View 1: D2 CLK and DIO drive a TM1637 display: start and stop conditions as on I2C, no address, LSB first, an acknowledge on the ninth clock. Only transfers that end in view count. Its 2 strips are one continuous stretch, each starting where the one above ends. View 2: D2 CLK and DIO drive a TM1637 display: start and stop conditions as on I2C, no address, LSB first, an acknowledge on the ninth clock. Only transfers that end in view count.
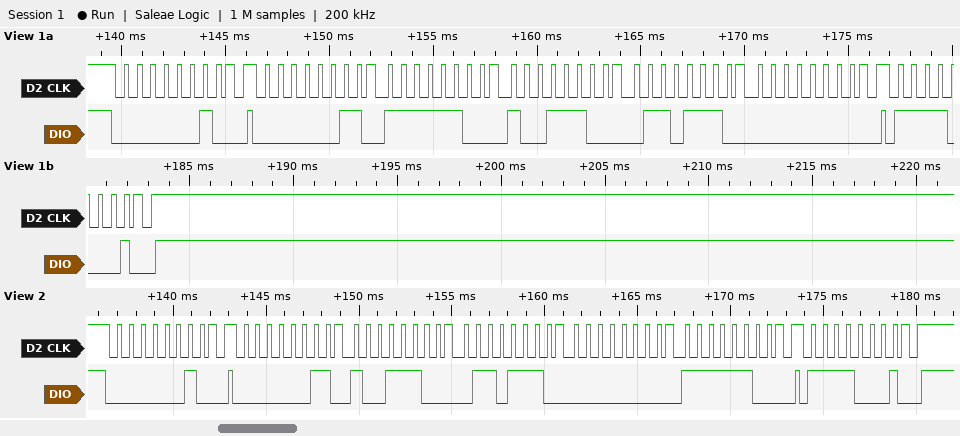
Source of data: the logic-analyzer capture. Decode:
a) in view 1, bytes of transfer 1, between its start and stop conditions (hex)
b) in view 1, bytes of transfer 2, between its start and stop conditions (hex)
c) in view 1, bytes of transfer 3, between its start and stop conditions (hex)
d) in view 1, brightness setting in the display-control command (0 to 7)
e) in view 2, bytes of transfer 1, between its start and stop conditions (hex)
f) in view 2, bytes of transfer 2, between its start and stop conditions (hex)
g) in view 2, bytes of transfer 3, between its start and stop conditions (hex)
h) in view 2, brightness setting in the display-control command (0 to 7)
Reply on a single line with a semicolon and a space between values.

40; C0 3F 39 76 00; 8F; 7; 40; C0 39 76 00 3F; 8F; 7
